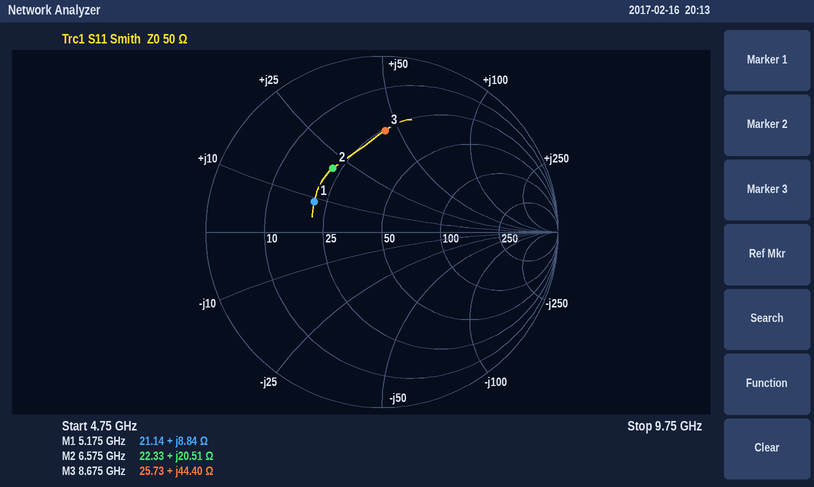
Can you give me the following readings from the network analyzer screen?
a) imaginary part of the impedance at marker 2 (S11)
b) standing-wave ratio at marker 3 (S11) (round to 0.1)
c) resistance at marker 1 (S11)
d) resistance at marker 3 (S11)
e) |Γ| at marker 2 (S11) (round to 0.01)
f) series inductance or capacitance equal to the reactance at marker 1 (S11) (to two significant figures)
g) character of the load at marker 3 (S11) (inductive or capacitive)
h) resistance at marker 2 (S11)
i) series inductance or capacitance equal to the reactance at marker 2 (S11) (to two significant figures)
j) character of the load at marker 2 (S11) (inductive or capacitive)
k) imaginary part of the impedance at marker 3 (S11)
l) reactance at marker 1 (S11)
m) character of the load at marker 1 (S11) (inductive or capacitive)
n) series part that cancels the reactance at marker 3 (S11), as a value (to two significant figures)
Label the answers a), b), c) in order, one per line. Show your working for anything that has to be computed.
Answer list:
a) +20.51 Ω
b) 3.7
c) 21.14 Ω
d) 25.73 Ω
e) 0.46
f) L = 8.84 Ω/(2π × 5.175 GHz) ≈ 272 pH, so 270 pH to two significant figures
g) inductive
h) 22.33 Ω
i) L = 20.51 Ω/(2π × 6.575 GHz) ≈ 496 pH, so 500 pH to two significant figures
j) inductive
k) +44.40 Ω
l) +8.84 Ω
m) inductive
n) C = 1/(2π × 8.675 GHz × 44.4 Ω) ≈ 413 fF, so 410 fF to two significant figures
